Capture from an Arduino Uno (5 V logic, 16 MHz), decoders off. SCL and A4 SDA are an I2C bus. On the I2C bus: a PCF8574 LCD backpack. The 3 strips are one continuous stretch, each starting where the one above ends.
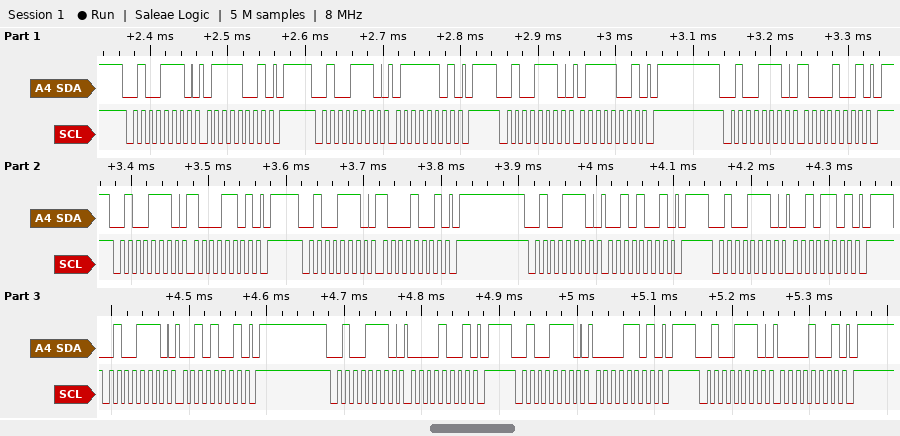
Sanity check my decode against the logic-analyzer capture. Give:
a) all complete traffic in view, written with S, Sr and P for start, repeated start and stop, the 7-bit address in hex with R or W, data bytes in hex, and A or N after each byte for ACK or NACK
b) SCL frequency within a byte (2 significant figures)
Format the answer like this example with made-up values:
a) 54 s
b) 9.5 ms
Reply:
a) S 27W A 79 A P S 27W A 7D A P S 27W A 79 A P S 27W A 89 A P S 27W A 8D A P S 27W A 89 A P S 27W A 29 A P S 27W A 2D A P S 27W A 29 A P S 27W A 09 A P S 27W A 0D A P S 27W A 09 A P
b) 100 kHz
